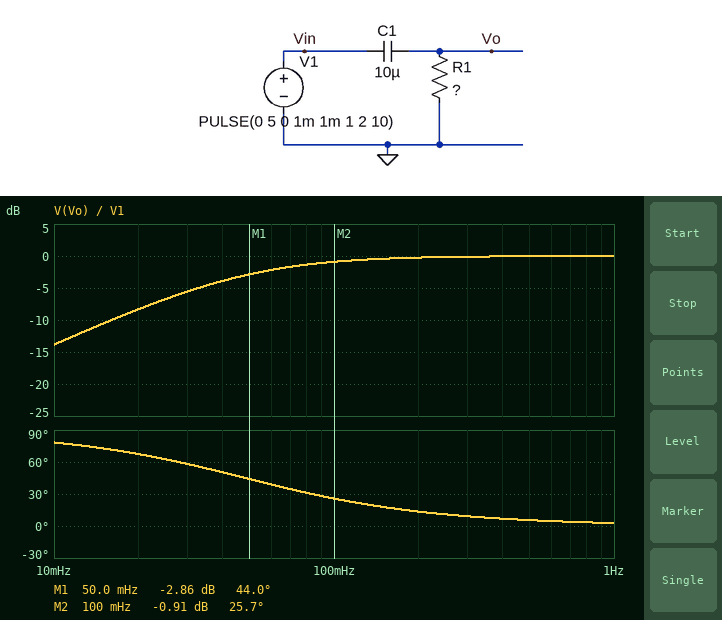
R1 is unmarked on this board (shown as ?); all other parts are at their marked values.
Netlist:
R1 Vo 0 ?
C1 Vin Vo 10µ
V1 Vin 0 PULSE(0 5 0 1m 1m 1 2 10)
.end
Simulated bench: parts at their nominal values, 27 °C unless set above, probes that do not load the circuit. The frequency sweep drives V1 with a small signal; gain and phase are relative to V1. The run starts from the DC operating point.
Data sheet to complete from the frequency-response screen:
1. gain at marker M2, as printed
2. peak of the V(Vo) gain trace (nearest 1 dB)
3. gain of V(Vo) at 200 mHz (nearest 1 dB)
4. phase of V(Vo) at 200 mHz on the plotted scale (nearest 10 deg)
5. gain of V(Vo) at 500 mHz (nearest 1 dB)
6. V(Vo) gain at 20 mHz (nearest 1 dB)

-0.91 dB
0 dB
0 dB
10 deg
0 dB
-8 dB
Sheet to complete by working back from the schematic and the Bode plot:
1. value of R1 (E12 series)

330 kΩ
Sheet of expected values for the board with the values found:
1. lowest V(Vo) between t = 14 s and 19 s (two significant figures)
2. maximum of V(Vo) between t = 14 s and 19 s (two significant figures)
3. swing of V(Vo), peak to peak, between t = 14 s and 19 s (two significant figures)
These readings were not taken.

-2.9 V
2.9 V
5.8 V
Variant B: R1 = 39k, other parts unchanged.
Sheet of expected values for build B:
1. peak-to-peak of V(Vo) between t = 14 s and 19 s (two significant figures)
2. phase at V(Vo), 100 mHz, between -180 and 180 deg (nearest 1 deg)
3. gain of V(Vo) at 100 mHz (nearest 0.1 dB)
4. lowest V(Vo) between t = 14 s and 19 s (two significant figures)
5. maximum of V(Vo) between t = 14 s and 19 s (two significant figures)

9.3 V
76 deg
-12.5 dB
-4.6 V
4.6 V
